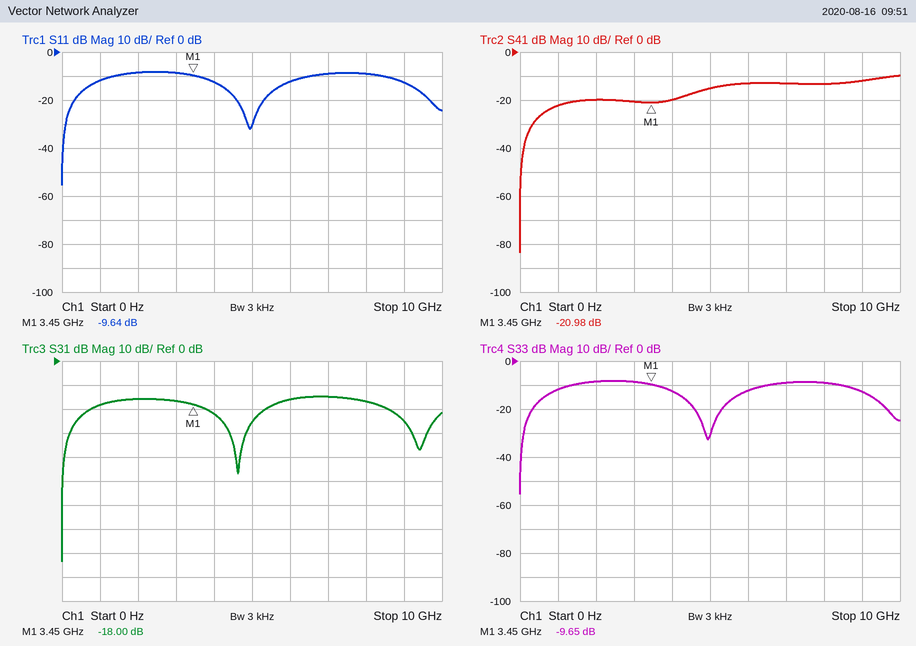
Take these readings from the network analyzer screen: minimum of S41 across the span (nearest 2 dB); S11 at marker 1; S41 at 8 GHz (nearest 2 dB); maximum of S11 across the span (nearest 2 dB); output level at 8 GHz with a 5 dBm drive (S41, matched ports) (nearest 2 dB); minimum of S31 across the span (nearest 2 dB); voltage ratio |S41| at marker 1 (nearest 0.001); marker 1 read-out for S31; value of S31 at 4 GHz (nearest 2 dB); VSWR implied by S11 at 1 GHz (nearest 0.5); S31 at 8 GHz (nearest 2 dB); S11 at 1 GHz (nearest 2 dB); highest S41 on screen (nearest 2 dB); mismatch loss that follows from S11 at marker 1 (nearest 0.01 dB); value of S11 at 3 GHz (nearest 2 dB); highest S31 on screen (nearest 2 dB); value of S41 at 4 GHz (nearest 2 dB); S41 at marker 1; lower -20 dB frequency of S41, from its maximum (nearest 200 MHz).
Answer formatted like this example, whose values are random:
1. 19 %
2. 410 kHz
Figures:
1. -84 dB
2. -9.64 dB
3. -14 dB
4. -8 dB
5. -8 dBm
6. -84 dB
7. 0.089
8. -18.00 dB
9. -22 dB
10. 1.5
11. -16 dB
12. -12 dB
13. -10 dB
14. 0.50 dB
15. -8 dB
16. -14 dB
17. -20 dB
18. -20.98 dB
19. 400 MHz
